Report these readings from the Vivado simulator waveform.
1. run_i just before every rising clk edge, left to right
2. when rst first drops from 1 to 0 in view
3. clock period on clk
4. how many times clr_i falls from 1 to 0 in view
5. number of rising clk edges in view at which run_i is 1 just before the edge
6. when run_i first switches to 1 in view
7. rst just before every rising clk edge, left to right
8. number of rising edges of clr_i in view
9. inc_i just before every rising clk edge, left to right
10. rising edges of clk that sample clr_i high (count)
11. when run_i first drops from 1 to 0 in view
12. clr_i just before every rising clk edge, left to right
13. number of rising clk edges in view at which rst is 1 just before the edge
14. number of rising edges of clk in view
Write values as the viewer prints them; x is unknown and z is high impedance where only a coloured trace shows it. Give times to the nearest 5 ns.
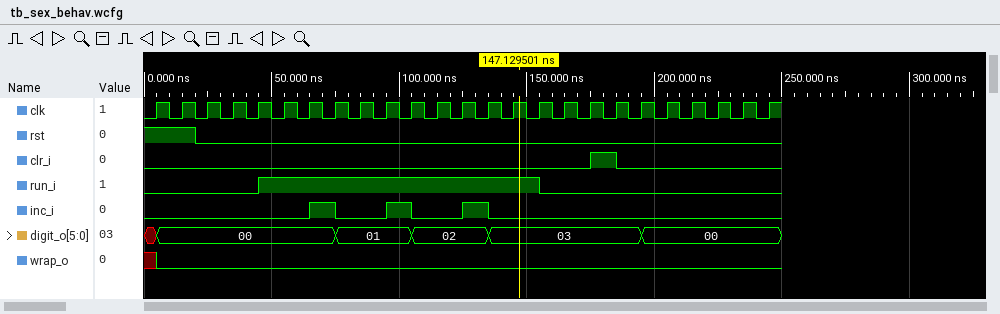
0 0 0 0 0 1 1 1 1 1 1 1 1 1 1 1 0 0 0 0 0 0 0 0 0
20 ns
10 ns
1
11
45 ns
1 1 0 0 0 0 0 0 0 0 0 0 0 0 0 0 0 0 0 0 0 0 0 0 0
1
0 0 0 0 0 0 0 1 0 0 1 0 0 1 0 0 0 0 0 0 0 0 0 0 0
1
155 ns
0 0 0 0 0 0 0 0 0 0 0 0 0 0 0 0 0 0 1 0 0 0 0 0 0
2
25
